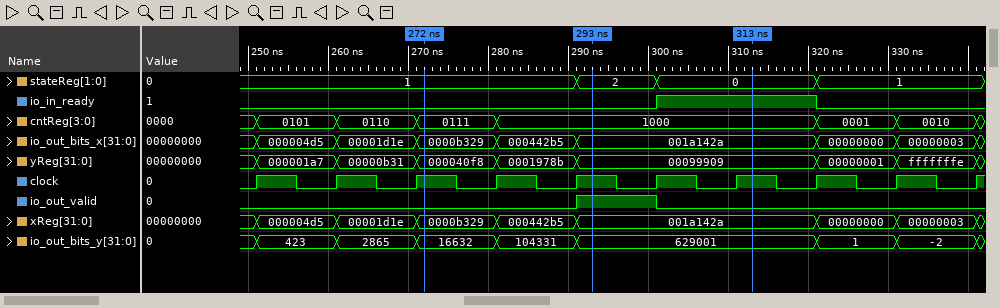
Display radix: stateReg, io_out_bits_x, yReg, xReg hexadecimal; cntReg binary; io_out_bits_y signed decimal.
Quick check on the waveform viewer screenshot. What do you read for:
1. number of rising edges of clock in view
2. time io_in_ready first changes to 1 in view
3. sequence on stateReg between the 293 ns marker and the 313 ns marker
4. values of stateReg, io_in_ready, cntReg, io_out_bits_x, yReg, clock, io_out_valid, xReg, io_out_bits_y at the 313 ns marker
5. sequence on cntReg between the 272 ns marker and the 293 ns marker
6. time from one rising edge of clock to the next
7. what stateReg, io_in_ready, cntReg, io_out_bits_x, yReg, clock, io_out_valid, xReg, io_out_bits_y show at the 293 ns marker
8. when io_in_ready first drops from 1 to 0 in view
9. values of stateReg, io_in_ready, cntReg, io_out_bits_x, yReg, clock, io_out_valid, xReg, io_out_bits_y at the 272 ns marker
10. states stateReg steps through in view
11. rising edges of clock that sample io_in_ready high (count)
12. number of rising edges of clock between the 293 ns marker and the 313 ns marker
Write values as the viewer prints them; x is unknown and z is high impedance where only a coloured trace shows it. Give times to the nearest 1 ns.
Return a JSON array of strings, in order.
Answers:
["10", "301 ns", "2, 0", "stateReg=0, io_in_ready=1, cntReg=1000, io_out_bits_x=001a142a, yReg=00099909, clock=1, io_out_valid=0, xReg=001a142a, io_out_bits_y=629001", "0111, 1000", "10 ns", "stateReg=2, io_in_ready=0, cntReg=1000, io_out_bits_x=001a142a, yReg=00099909, clock=1, io_out_valid=1, xReg=001a142a, io_out_bits_y=629001", "321 ns", "stateReg=1, io_in_ready=0, cntReg=0111, io_out_bits_x=0000b329, yReg=000040f8, clock=1, io_out_valid=0, xReg=0000b329, io_out_bits_y=16632", "1, 2, 0, 1", "2", "2"]
